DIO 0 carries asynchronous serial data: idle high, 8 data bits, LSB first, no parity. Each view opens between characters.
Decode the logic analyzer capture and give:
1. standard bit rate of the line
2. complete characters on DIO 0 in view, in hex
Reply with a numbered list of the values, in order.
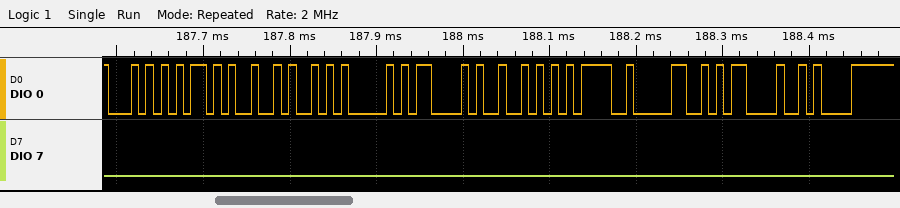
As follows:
1. 115200 baud
2. 54, 2B, 4A, 41, 43, 52, 3D, 30, 0D, 0A
